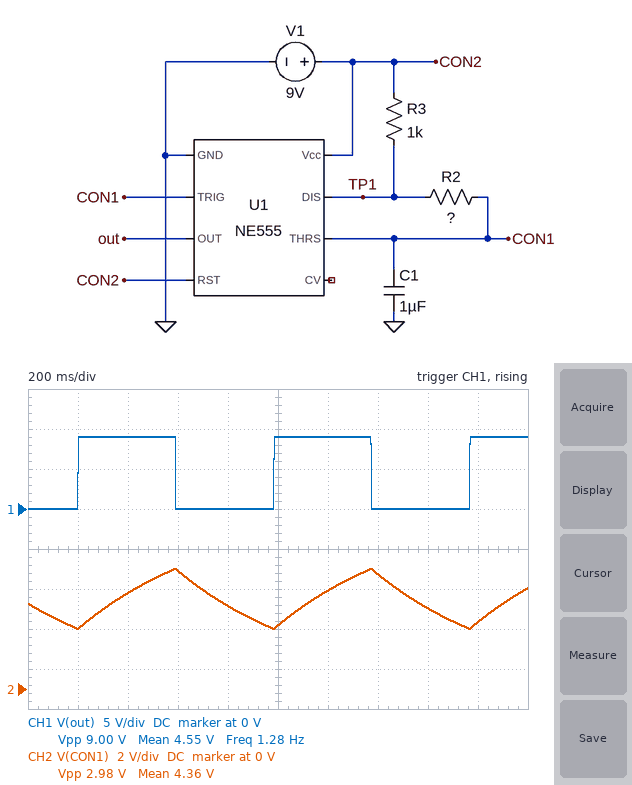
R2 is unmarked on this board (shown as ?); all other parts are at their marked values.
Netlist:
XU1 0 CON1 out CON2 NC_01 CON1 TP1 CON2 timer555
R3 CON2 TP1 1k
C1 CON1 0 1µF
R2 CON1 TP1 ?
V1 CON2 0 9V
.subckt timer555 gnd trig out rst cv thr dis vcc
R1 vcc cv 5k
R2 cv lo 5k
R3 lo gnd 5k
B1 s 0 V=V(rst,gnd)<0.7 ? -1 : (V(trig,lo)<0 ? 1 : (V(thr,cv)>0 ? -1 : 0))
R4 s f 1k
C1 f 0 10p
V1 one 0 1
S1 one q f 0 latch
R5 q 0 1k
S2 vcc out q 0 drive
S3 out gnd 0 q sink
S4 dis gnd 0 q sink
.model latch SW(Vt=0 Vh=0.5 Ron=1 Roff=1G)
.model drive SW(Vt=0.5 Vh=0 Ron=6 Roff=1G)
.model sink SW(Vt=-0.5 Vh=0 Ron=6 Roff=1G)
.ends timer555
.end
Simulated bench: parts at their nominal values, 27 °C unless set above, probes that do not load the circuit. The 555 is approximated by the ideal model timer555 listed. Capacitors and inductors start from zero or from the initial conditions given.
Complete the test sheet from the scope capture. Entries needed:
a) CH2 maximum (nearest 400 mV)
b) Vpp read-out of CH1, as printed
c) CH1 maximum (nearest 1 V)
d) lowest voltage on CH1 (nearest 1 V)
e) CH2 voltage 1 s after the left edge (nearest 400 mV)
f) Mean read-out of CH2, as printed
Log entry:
6.0 V
9.00 V
9 V
0 V
3.2 V
4.36 V
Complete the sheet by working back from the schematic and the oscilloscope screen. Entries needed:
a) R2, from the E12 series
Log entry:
560 kΩ
